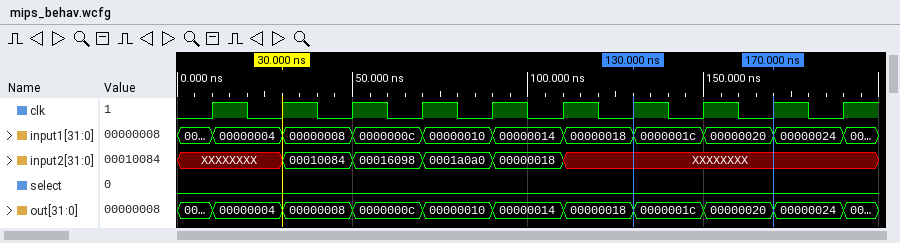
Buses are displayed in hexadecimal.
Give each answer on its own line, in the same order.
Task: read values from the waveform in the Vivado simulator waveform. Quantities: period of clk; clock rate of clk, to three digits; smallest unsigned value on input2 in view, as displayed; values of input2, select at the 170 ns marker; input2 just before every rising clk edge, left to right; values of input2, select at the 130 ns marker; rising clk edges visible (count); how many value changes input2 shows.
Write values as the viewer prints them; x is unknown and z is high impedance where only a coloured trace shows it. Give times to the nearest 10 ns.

20 ns
50.0 MHz
00000018
input2=XXXXXXXX, select=0
XXXXXXXX, XXXXXXXX, 00010084, 00016098, 0001a0a0, 00000018, XXXXXXXX, XXXXXXXX, XXXXXXXX, XXXXXXXX
input2=XXXXXXXX, select=0
10
5
